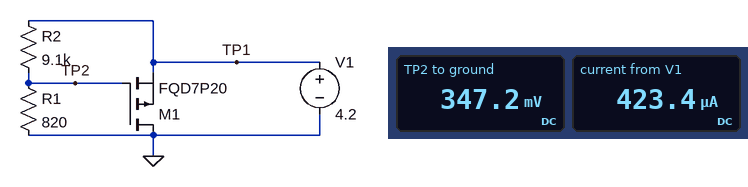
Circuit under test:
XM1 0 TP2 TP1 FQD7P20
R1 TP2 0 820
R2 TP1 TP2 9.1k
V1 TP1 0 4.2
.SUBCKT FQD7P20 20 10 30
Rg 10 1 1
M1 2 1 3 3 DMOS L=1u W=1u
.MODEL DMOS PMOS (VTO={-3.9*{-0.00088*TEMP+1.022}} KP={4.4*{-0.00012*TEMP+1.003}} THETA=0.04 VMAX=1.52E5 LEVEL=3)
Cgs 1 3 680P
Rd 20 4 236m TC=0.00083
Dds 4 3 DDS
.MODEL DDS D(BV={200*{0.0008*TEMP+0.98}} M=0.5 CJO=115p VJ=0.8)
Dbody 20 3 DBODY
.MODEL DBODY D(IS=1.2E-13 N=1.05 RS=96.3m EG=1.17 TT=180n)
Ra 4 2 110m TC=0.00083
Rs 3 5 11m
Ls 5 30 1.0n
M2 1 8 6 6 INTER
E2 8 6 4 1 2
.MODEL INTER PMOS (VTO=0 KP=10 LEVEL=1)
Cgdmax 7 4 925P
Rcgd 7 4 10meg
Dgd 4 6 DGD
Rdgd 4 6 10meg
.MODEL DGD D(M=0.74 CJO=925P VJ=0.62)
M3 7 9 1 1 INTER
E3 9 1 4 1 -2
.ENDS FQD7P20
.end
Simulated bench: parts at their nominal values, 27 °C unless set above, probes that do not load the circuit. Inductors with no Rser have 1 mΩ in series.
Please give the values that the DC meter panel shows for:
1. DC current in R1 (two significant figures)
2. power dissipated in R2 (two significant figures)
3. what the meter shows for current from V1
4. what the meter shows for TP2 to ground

420 µA
1.6 mW
423.4 µA
347.2 mV
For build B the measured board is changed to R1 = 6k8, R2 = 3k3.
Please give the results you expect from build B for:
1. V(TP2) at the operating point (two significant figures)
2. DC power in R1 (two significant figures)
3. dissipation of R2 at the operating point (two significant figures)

2.8 V
1.2 mW
570 µW
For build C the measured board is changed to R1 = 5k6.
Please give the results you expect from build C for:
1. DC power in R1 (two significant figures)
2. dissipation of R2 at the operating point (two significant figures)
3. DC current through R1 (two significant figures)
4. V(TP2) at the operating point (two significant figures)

460 µW
740 µW
290 µA
1.6 V
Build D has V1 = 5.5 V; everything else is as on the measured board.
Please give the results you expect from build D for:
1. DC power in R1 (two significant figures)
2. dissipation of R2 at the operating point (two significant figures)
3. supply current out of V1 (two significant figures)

250 µW
2.8 mW
1.9 A
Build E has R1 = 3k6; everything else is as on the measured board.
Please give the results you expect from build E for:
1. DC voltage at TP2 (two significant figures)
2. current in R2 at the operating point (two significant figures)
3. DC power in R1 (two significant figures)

1.2 V
330 µA
390 µW
